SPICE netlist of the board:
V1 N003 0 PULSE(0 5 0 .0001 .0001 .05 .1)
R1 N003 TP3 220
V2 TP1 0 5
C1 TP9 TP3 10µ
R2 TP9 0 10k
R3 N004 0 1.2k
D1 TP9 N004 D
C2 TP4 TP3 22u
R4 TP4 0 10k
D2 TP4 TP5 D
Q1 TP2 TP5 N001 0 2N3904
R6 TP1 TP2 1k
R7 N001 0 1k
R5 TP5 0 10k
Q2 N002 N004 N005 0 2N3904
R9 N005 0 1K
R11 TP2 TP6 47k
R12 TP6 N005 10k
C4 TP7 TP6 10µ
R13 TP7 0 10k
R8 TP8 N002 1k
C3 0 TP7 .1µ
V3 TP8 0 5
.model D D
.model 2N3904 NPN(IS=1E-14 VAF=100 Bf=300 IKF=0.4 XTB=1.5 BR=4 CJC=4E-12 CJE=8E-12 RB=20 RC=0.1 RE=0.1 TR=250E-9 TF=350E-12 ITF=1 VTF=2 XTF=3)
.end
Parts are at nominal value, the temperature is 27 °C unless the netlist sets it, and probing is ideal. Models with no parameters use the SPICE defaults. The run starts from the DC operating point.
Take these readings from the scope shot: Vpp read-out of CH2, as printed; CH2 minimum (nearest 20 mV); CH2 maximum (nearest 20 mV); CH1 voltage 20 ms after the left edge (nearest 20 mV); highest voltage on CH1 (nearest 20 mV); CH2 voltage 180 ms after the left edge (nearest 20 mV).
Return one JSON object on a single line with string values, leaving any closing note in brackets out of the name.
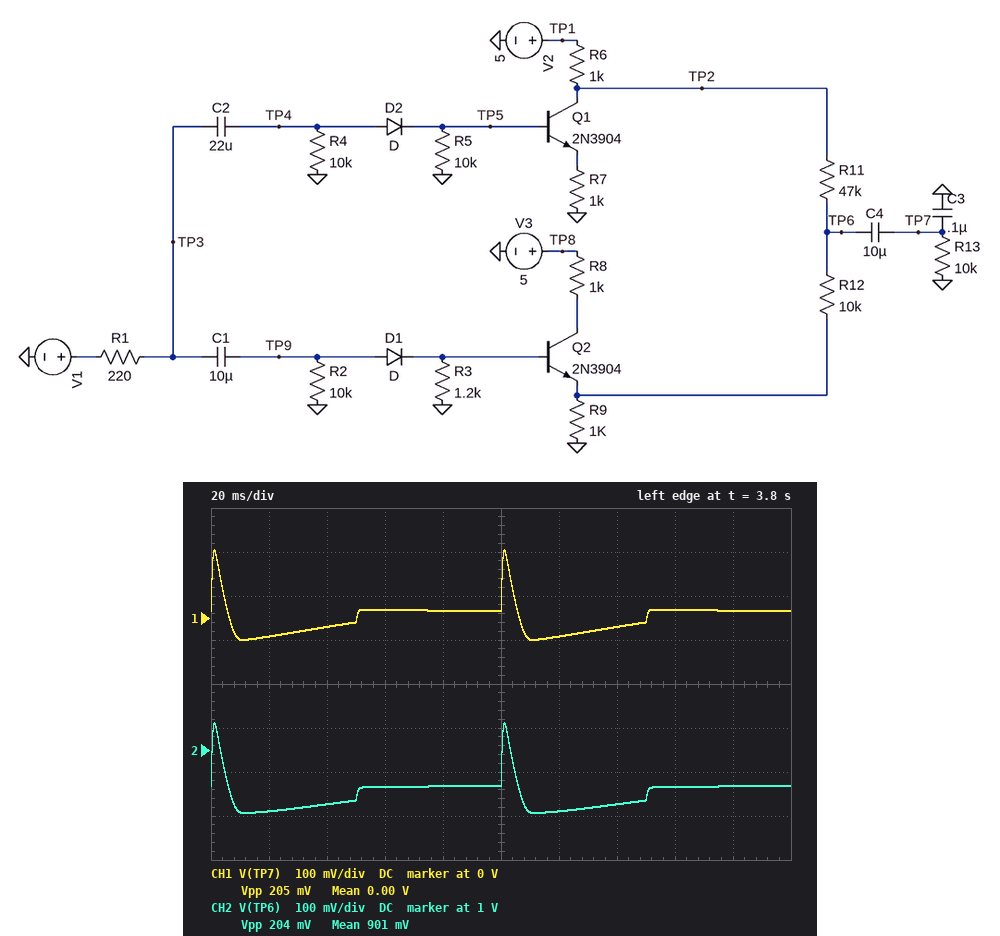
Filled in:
{"Vpp read-out of CH2, as printed": "204 mV", "CH2 minimum": "860 mV", "CH2 maximum": "1.06 V", "CH1 voltage 20 ms after the left edge": "-40 mV", "highest voltage on CH1": "160 mV", "CH2 voltage 180 ms after the left edge": "920 mV"}
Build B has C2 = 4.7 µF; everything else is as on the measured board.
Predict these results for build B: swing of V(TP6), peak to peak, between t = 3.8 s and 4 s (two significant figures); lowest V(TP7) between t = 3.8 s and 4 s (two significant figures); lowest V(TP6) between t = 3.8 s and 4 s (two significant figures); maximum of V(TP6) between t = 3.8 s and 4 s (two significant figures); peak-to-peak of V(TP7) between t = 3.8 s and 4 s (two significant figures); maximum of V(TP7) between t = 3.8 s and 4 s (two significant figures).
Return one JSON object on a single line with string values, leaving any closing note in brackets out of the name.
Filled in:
{"swing of V(TP6), peak to peak, between t = 3.8 s and 4 s": "140 mV", "lowest V(TP7) between t = 3.8 s and 4 s": "-86 mV", "lowest V(TP6) between t = 3.8 s and 4 s": "820 mV", "maximum of V(TP6) between t = 3.8 s and 4 s": "960 mV", "peak-to-peak of V(TP7) between t = 3.8 s and 4 s": "130 mV", "maximum of V(TP7) between t = 3.8 s and 4 s": "46 mV"}
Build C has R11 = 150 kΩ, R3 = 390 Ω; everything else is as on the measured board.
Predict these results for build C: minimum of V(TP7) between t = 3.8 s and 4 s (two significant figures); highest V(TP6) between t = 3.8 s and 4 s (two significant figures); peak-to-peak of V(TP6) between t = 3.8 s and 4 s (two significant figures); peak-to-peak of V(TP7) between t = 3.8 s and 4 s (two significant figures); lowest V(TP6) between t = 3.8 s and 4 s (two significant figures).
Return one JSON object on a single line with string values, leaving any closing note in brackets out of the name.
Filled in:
{"minimum of V(TP7) between t = 3.8 s and 4 s": "-16 mV", "highest V(TP6) between t = 3.8 s and 4 s": "400 mV", "peak-to-peak of V(TP6) between t = 3.8 s and 4 s": "93 mV", "peak-to-peak of V(TP7) between t = 3.8 s and 4 s": "92 mV", "lowest V(TP6) between t = 3.8 s and 4 s": "310 mV"}
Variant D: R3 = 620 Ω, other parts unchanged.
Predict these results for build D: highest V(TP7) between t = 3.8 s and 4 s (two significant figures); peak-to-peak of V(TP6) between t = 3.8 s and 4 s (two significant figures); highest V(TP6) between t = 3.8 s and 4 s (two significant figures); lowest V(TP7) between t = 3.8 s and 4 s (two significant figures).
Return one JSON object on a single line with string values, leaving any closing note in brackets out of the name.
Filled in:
{"highest V(TP7) between t = 3.8 s and 4 s": "92 mV", "peak-to-peak of V(TP6) between t = 3.8 s and 4 s": "140 mV", "highest V(TP6) between t = 3.8 s and 4 s": "990 mV", "lowest V(TP7) between t = 3.8 s and 4 s": "-44 mV"}
